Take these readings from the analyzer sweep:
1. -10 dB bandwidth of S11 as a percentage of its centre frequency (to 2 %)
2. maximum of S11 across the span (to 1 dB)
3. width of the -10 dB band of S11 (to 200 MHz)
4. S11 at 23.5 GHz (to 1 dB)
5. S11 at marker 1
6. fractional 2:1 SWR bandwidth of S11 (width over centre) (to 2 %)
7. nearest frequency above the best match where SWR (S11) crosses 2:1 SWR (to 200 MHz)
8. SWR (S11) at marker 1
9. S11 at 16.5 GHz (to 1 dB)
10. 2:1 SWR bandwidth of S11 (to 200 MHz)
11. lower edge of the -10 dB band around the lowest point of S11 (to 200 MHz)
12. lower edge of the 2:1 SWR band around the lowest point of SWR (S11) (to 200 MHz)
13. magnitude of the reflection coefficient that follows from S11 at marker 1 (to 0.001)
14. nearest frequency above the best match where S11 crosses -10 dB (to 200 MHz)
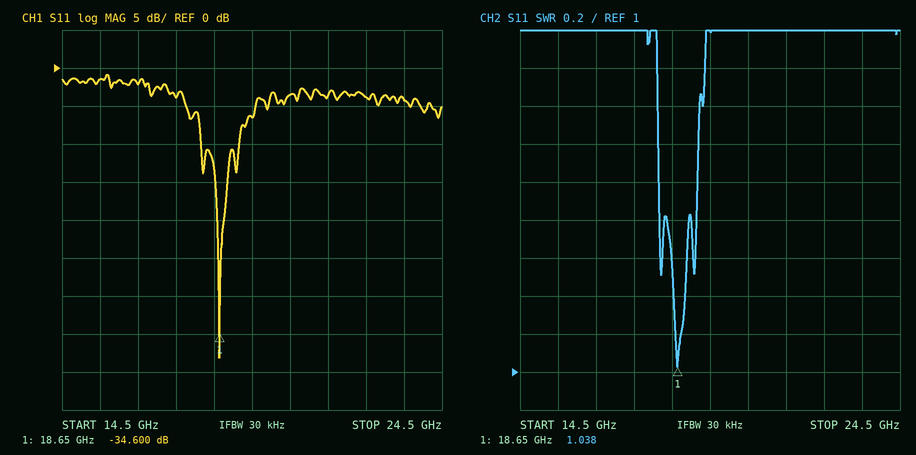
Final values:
6 %
-1 dB
1.0 GHz
-4 dB
-34.600 dB
6 %
19.2 GHz
1.038
-2 dB
1.0 GHz
18.2 GHz
18.2 GHz
0.019
19.2 GHz
